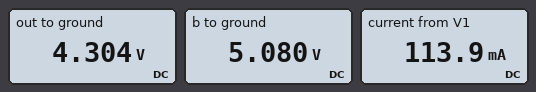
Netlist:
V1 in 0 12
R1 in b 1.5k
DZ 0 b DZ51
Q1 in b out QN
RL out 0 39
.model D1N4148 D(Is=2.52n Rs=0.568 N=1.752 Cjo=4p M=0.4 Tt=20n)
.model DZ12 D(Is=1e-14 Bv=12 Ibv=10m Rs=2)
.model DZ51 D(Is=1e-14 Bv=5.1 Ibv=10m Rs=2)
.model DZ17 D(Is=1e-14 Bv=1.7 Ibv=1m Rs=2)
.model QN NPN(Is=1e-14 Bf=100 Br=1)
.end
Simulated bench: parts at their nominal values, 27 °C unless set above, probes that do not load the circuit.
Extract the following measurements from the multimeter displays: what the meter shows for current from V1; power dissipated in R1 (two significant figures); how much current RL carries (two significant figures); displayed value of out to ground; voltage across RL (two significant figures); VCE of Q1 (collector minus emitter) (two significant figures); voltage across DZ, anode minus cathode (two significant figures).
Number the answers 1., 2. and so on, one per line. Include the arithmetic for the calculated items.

1. 113.9 mA
2. (12 V - 5.08 V)^2 / 1.5 kΩ = 32 mW
3. (4.304 V) / 39 Ω = 110 mA
4. 4.304 V
5. 4.304 V = 4.3 V
6. 12 V - 4.304 V = 7.7 V
7. 0 V - 5.08 V = -5.1 V
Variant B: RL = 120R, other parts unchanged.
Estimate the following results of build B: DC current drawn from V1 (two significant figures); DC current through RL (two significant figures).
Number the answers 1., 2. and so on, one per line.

1. 40 mA
2. 36 mA
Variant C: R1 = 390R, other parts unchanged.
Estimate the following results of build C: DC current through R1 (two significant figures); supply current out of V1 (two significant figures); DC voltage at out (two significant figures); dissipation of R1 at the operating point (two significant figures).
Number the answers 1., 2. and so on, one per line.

1. 18 mA
2. 130 mA
3. 4.4 V
4. 120 mW
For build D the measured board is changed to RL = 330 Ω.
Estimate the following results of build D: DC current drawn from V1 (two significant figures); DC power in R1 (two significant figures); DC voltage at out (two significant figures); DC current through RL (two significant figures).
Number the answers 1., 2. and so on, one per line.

1. 18 mA
2. 32 mW
3. 4.4 V
4. 13 mA
